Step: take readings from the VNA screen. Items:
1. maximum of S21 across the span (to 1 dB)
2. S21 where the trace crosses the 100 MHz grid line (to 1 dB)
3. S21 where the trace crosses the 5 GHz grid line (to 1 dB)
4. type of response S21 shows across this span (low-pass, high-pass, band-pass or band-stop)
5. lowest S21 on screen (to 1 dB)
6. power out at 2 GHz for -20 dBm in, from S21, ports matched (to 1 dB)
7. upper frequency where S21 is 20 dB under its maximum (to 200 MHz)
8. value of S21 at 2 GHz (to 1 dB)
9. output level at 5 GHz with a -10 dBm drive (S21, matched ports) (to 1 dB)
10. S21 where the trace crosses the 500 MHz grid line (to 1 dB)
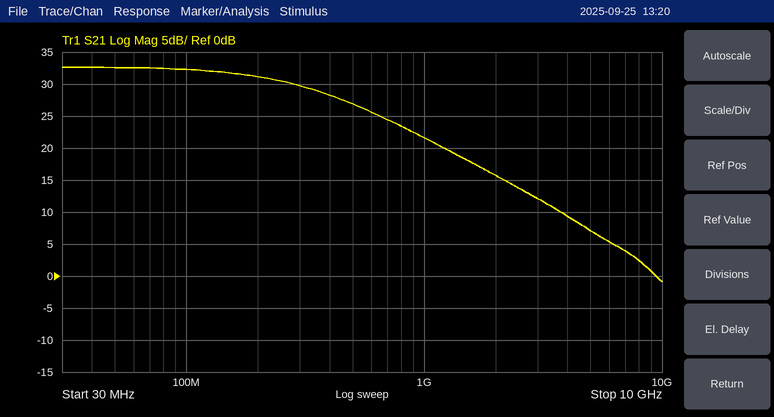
33 dB
32 dB
7 dB
low-pass
-1 dB
-4 dBm
2.8 GHz
16 dB
-3 dBm
27 dB
